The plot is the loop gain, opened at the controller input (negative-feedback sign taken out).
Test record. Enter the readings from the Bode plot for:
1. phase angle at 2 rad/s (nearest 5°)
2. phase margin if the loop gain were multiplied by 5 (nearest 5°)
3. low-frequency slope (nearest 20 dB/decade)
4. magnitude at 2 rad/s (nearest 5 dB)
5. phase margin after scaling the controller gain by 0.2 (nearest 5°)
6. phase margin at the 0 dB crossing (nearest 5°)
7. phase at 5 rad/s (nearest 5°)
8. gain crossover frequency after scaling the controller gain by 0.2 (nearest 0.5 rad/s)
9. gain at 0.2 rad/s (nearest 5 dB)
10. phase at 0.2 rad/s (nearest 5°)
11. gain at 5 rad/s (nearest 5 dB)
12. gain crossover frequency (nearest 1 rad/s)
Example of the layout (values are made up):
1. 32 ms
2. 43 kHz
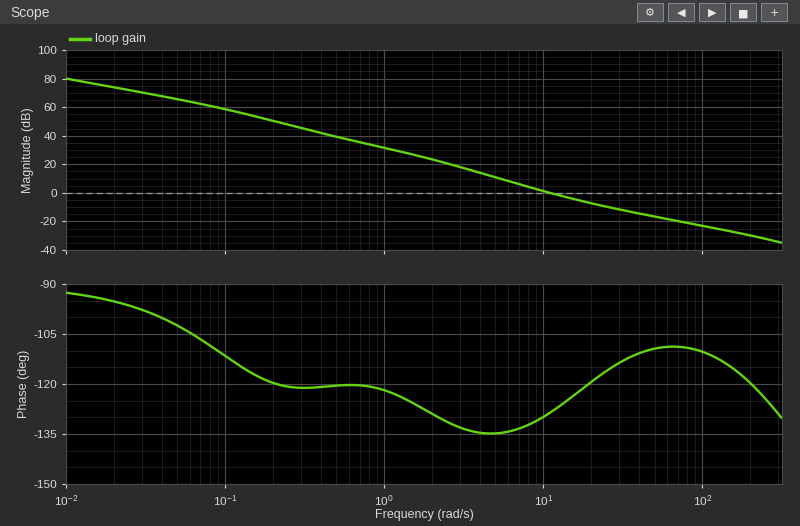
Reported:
1. -130°
2. 70°
3. -20 dB/decade
4. 25 dB
5. 45°
6. 50°
7. -135°
8. 4.0 rad/s
9. 50 dB
10. -120°
11. 10 dB
12. 11 rad/s
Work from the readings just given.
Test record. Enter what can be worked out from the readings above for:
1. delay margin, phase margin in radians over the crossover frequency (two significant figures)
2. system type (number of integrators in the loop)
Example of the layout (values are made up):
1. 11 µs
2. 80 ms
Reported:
1. 0.079 s
2. 1
